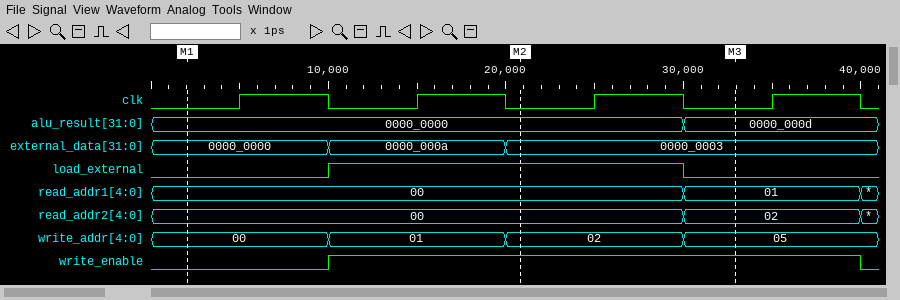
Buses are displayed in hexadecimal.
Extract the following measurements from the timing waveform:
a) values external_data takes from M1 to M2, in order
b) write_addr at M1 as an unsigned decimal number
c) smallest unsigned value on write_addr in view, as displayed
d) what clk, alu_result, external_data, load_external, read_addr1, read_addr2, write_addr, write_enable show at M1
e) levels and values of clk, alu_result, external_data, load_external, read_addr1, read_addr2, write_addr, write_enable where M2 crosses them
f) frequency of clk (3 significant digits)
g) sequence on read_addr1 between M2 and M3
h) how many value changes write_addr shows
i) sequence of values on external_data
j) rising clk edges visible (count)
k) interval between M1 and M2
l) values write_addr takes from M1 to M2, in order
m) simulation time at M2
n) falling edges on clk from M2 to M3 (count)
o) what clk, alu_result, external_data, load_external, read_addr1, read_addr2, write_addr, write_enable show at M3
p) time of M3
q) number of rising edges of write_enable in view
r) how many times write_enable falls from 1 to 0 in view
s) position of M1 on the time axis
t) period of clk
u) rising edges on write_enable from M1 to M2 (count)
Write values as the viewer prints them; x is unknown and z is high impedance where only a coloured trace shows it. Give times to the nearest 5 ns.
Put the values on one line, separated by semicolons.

0000_0000, 0000_000a, 0000_0003; 0; 00; clk=0, alu_result=0000_0000, external_data=0000_0000, load_external=0, read_addr1=00, read_addr2=00, write_addr=00, write_enable=0; clk=0, alu_result=0000_0000, external_data=0000_0003, load_external=1, read_addr1=00, read_addr2=00, write_addr=02, write_enable=1; 100 MHz; 00, 01; 3; 0000_0000, 0000_000a, 0000_0003; 4; 20 ns; 00, 01, 02; 20 ns; 1; clk=0, alu_result=0000_000d, external_data=0000_0003, load_external=0, read_addr1=01, read_addr2=02, write_addr=05, write_enable=1; 35 ns; 1; 1; 0 ns; 10 ns; 1
